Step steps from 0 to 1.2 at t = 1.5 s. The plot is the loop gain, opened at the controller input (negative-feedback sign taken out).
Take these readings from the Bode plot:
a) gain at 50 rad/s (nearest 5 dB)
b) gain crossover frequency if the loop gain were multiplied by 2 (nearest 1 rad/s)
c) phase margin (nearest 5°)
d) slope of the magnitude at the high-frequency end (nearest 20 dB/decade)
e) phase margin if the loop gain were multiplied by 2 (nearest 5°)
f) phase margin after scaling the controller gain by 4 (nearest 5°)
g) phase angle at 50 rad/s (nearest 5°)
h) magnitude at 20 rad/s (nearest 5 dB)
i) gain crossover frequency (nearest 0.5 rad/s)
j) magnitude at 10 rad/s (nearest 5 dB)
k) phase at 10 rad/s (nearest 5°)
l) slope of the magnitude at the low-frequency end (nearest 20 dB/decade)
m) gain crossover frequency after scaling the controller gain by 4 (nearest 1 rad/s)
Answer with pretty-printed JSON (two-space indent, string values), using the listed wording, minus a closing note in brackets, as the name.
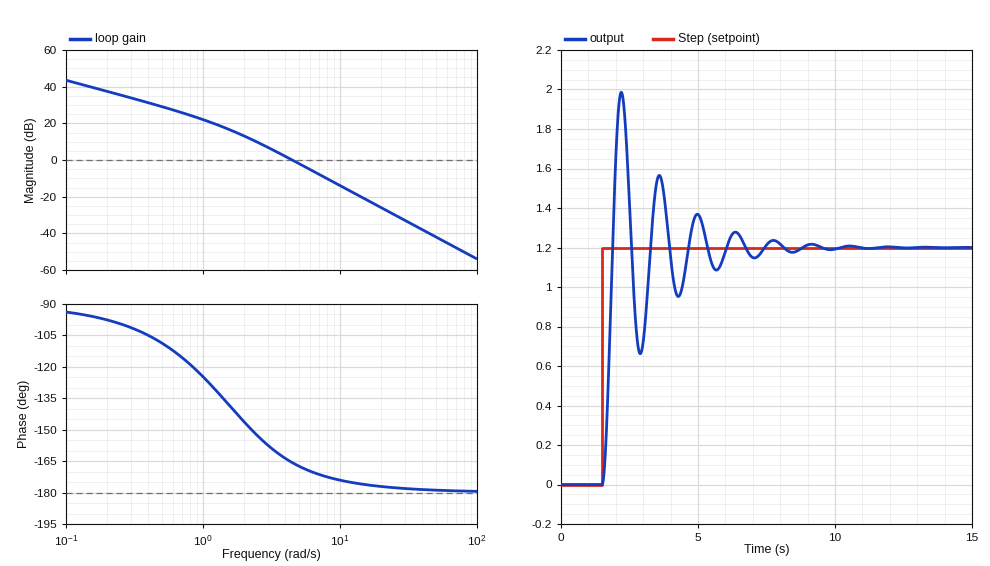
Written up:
{
  "gain at 50 rad/s": "-40 dB",
  "gain crossover frequency if the loop gain were multiplied by 2": "6 rad/s",
  "phase margin": "15°",
  "slope of the magnitude at the high-frequency end": "-40 dB/decade",
  "phase margin if the loop gain were multiplied by 2": "10°",
  "phase margin after scaling the controller gain by 4": "5°",
  "phase angle at 50 rad/s": "-180°",
  "magnitude at 20 rad/s": "-25 dB",
  "gain crossover frequency": "4.5 rad/s",
  "magnitude at 10 rad/s": "-15 dB",
  "phase at 10 rad/s": "-175°",
  "slope of the magnitude at the low-frequency end": "-20 dB/decade",
  "gain crossover frequency after scaling the controller gain by 4": "9 rad/s"
}
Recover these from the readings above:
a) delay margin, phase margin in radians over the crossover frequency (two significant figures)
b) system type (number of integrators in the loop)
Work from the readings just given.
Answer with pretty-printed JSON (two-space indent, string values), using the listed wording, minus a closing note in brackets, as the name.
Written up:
{
  "delay margin, phase margin in radians over the crossover frequency": "0.058 s",
  "system type": "1"
}
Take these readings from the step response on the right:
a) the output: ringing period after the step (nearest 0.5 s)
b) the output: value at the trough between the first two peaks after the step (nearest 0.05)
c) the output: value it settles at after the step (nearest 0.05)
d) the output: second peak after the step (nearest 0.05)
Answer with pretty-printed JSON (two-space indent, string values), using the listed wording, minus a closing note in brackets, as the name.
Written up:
{
  "the output: ringing period after the step": "1.5 s",
  "the output: value at the trough between the first two peaks after the step": "0.65",
  "the output: value it settles at after the step": "1.20",
  "the output: second peak after the step": "1.55"
}
